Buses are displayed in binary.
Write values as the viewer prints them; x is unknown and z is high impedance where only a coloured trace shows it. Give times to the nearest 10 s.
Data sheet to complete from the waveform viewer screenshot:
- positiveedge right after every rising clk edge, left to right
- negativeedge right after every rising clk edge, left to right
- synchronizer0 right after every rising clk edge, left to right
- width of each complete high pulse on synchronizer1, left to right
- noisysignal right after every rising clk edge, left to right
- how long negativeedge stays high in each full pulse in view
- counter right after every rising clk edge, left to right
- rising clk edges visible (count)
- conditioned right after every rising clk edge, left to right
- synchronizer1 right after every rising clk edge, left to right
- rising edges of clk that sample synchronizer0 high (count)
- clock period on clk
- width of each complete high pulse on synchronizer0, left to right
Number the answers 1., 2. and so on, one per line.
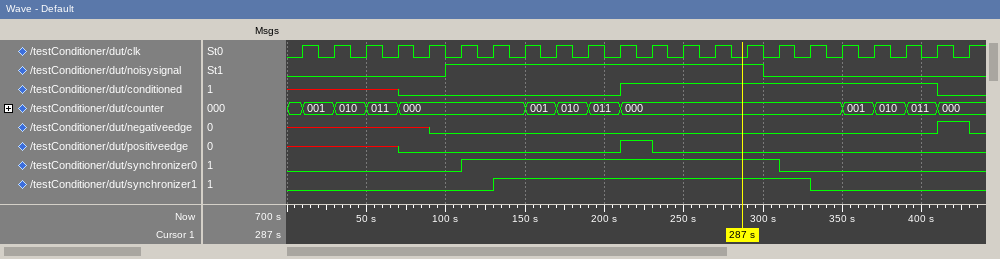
1. x x x 0 0 0 0 0 0 0 1 0 0 0 0 0 0 0 0 0 0 0
2. x x x x 0 0 0 0 0 0 0 0 0 0 0 0 0 0 0 0 1 0
3. 0 0 0 0 0 1 1 1 1 1 1 1 1 1 1 0 0 0 0 0 0 0
4. 200 s
5. 0 0 0 0 0 1 1 1 1 1 1 1 1 1 1 0 0 0 0 0 0 0
6. 20 s
7. 001, 010, 011, 000, 000, 000, 000, 001, 010, 011, 000, 000, 000, 000, 000, 000, 000, 001, 010, 011, 000, 000
8. 22
9. x x x 0 0 0 0 0 0 0 1 1 1 1 1 1 1 1 1 1 0 0
10. 0 0 0 0 0 0 1 1 1 1 1 1 1 1 1 1 0 0 0 0 0 0
11. 10
12. 20 s
13. 200 s
